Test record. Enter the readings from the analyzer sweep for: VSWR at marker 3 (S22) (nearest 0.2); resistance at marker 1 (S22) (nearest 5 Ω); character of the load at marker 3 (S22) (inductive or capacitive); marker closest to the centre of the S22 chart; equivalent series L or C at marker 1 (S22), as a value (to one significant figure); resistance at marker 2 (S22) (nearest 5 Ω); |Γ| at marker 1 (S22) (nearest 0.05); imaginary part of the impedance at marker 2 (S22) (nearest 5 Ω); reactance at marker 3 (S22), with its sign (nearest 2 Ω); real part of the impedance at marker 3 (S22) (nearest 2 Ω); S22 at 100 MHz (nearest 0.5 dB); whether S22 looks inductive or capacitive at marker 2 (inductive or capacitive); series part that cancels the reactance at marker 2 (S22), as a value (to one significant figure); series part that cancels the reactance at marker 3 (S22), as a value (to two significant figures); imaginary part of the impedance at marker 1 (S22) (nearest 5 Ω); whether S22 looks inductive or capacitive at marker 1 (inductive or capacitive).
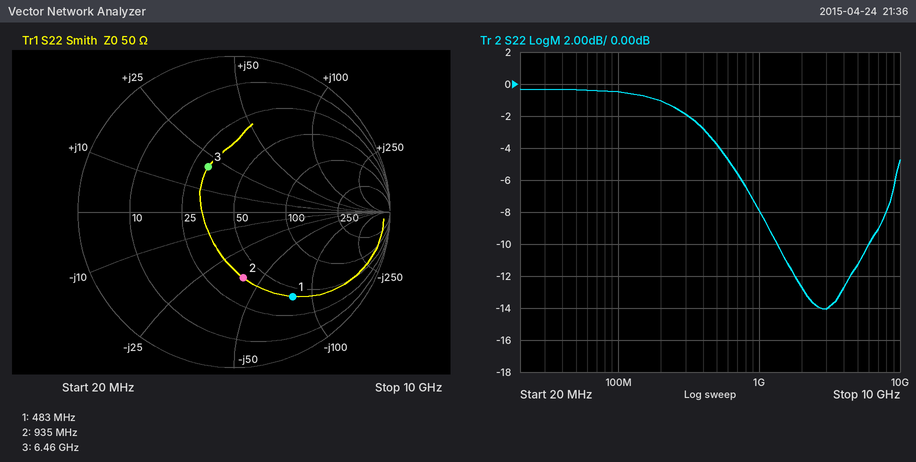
2.0
40 Ω
inductive
marker 3
4 pF
40 Ω
0.65
-40 Ω
+20 Ω
30 Ω
-0.5 dB
capacitive
7 nH
1.2 pF
-80 Ω
capacitive
